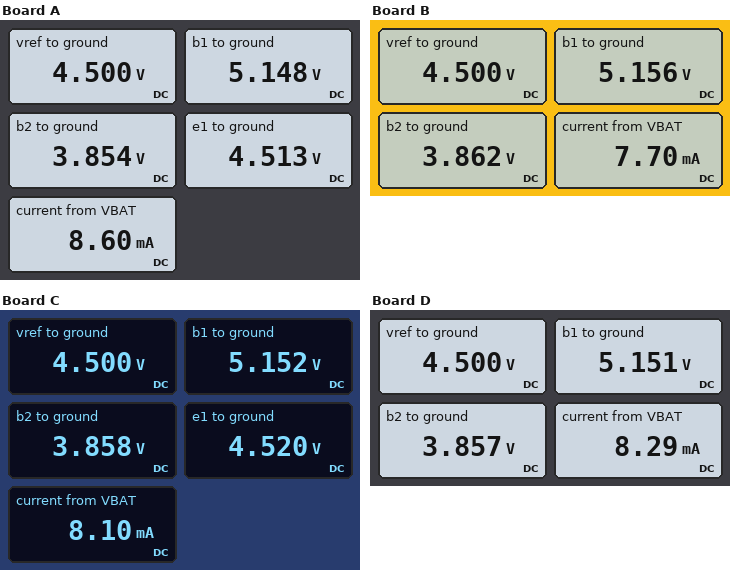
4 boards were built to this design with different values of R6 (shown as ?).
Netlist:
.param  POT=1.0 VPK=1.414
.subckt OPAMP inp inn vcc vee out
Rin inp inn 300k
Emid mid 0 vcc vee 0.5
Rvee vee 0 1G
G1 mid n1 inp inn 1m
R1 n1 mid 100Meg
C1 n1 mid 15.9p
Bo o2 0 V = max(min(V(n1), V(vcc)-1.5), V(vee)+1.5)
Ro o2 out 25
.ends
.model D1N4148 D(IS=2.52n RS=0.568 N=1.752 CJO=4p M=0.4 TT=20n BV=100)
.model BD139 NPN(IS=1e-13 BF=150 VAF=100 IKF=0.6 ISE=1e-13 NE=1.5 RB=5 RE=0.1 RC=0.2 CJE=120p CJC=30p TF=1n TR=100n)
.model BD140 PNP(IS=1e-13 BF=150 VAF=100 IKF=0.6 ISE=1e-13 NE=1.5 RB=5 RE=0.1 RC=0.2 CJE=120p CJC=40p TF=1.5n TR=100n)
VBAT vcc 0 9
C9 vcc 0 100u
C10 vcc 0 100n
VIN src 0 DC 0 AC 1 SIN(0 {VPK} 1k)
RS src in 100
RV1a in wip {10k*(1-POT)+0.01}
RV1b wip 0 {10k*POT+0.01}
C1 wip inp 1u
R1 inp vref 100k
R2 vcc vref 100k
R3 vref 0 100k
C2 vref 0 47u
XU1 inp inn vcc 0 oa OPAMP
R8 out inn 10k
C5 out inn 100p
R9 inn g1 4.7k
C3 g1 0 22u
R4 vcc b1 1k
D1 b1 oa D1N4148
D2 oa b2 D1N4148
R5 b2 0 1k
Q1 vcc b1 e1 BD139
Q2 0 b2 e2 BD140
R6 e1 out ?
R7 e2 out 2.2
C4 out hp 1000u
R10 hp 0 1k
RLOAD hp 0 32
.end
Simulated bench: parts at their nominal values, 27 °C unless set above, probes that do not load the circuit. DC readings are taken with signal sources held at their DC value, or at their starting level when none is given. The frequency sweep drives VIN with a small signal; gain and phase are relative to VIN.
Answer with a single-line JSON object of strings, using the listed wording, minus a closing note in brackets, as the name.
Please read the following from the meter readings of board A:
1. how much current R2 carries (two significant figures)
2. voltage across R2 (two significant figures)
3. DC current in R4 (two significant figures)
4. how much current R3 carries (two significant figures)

{"how much current R2 carries": "45 µA", "voltage across R2": "4.5 V", "DC current in R4": "3.9 mA", "how much current R3 carries": "45 µA"}
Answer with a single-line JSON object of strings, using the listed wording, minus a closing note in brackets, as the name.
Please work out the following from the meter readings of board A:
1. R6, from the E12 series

{"R6, from the E12 series": "2.7 Ω"}
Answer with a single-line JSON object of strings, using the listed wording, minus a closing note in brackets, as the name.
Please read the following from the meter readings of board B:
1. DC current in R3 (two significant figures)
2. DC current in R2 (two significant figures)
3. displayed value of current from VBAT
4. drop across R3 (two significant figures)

{"DC current in R3": "45 µA", "DC current in R2": "45 µA", "displayed value of current from VBAT": "7.70 mA", "drop across R3": "4.5 V"}
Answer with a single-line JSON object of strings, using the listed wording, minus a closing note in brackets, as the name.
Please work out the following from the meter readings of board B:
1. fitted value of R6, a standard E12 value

{"fitted value of R6, a standard E12 value": "6.8 Ω"}
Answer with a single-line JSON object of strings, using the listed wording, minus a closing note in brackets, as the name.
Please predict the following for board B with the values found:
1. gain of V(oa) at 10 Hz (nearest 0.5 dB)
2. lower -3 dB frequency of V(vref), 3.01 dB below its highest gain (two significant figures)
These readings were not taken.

{"gain of V(oa) at 10 Hz": "11.0 dB", "lower -3 dB frequency of V(vref), 3.01 dB below its highest gain": "61 mHz"}
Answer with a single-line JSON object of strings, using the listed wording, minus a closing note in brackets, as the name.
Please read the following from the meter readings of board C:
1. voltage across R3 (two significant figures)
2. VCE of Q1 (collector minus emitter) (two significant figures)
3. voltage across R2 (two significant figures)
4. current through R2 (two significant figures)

{"voltage across R3": "4.5 V", "VCE of Q1 (collector minus emitter)": "4.5 V", "voltage across R2": "4.5 V", "current through R2": "45 µA"}
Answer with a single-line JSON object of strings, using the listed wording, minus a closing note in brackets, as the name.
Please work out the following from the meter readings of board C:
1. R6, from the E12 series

{"R6, from the E12 series": "4.7 Ω"}
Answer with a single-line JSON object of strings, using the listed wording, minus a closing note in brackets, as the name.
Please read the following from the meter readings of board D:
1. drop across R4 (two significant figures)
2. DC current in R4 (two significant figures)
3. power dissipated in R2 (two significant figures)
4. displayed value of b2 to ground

{"drop across R4": "3.8 V", "DC current in R4": "3.8 mA", "power dissipated in R2": "200 µW", "displayed value of b2 to ground": "3.857 V"}
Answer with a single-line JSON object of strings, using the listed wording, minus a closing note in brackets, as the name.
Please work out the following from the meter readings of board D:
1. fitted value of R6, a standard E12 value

{"fitted value of R6, a standard E12 value": "3.9 Ω"}
